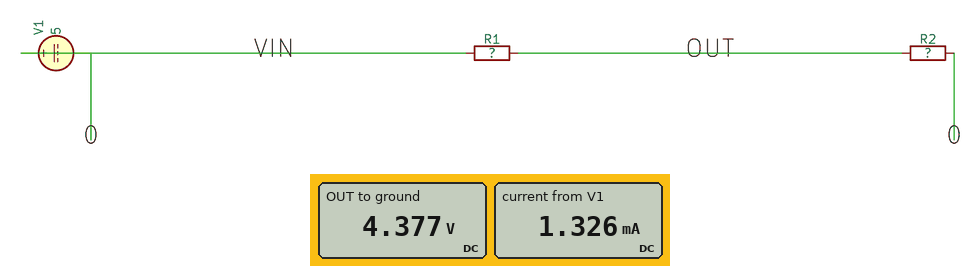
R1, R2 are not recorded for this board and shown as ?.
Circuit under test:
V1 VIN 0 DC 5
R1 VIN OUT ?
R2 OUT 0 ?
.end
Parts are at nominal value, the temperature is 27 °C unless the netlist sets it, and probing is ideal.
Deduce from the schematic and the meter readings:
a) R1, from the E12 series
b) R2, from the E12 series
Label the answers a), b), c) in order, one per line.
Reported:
a) 470 Ω
b) 3.3 kΩ
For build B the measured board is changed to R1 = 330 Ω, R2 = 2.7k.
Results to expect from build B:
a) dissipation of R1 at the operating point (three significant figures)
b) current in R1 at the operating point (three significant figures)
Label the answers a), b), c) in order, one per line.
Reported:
a) 899 µW
b) 1.65 mA
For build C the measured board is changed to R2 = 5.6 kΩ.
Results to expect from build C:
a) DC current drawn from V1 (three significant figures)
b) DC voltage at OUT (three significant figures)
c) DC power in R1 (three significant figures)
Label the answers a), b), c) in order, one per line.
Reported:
a) 824 µA
b) 4.61 V
c) 319 µW
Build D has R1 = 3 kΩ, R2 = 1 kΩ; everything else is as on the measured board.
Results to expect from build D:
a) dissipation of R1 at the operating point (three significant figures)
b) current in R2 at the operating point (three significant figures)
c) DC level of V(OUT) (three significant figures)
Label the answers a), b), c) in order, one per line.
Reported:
a) 4.69 mW
b) 1.25 mA
c) 1.25 V
